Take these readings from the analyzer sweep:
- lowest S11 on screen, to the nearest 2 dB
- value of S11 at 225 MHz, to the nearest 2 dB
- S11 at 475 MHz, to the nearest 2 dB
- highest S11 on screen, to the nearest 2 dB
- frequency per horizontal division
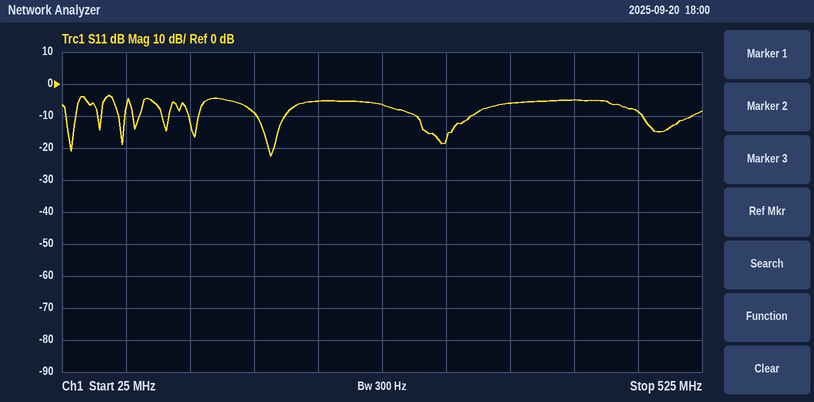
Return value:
-22 dB
-6 dB
-8 dB
-4 dB
50 MHz
